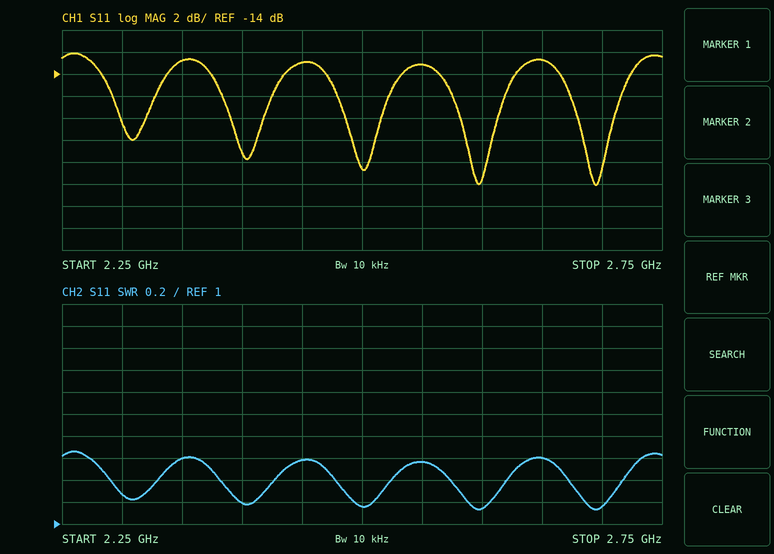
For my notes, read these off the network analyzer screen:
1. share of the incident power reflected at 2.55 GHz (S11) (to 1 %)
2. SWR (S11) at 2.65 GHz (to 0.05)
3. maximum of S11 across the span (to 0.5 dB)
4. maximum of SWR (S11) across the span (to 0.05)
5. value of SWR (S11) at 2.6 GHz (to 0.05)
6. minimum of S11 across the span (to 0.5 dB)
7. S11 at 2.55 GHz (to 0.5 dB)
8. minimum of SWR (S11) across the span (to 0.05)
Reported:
5 %
1.60
-12.0 dB
1.65
1.15
-24.0 dB
-13.0 dB
1.15
